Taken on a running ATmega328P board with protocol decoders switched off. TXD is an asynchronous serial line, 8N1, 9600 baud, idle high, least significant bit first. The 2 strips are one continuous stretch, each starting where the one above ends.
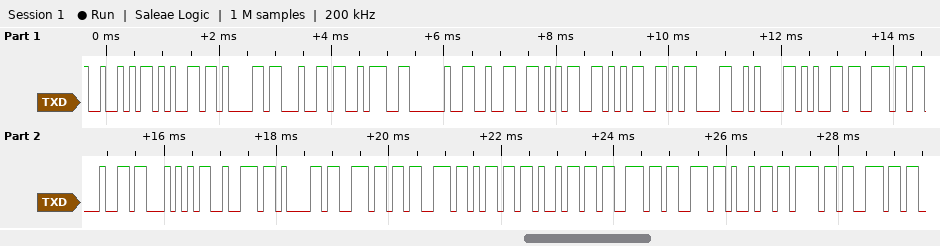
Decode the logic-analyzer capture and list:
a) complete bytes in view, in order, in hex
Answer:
52 65 61 64 3A 20 32 35 35 0D 0A 65 6E 64 54 72 61 6E 73 6D 69 73 73 69 6F 6E
